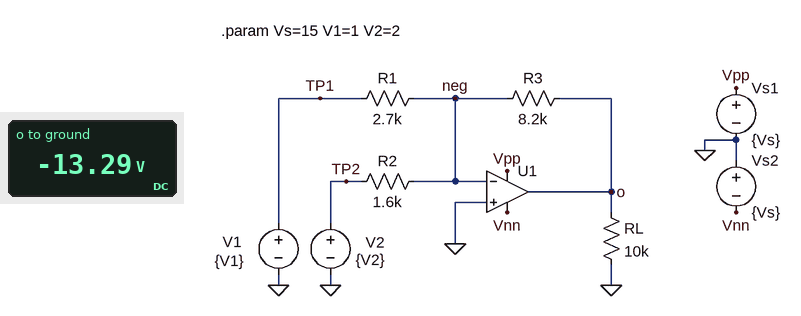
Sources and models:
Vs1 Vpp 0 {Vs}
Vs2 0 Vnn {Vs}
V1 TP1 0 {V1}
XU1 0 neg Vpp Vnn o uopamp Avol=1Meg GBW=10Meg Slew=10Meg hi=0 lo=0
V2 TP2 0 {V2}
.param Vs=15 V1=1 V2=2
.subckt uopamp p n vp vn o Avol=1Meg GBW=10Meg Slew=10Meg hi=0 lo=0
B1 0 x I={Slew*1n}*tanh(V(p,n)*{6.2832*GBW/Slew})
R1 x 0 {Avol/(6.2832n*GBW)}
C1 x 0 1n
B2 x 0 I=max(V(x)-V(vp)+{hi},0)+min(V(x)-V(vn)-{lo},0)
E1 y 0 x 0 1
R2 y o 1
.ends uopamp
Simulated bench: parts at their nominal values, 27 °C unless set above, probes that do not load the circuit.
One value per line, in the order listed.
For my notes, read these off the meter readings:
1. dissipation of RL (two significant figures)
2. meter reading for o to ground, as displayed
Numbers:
18 mW
-13.29 V
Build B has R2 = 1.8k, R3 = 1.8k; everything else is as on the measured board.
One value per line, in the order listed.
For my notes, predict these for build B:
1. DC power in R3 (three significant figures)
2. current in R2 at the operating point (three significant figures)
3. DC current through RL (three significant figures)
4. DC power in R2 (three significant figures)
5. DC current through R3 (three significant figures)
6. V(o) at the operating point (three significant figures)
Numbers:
3.95 mW
1.11 mA
267 µA
2.22 mW
1.48 mA
-2.67 V
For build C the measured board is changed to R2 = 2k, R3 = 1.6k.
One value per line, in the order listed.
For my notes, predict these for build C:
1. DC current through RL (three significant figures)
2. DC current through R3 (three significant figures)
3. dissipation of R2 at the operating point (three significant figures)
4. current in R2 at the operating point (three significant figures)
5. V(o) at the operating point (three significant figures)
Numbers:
219 µA
1.37 mA
2.00 mW
1.00 mA
-2.19 V
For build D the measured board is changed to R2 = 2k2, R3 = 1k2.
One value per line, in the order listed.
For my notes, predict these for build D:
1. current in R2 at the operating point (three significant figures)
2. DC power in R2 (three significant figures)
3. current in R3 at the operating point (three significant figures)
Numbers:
909 µA
1.82 mW
1.28 mA
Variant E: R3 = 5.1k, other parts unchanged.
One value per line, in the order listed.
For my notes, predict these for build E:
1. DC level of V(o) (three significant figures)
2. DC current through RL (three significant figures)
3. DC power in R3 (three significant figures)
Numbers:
-8.26 V
826 µA
13.4 mW
